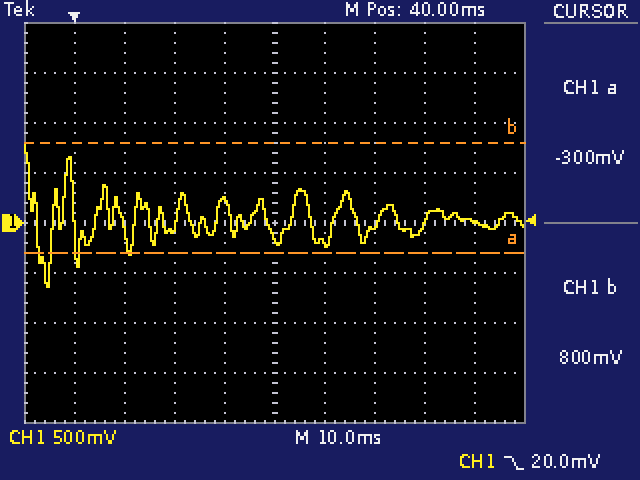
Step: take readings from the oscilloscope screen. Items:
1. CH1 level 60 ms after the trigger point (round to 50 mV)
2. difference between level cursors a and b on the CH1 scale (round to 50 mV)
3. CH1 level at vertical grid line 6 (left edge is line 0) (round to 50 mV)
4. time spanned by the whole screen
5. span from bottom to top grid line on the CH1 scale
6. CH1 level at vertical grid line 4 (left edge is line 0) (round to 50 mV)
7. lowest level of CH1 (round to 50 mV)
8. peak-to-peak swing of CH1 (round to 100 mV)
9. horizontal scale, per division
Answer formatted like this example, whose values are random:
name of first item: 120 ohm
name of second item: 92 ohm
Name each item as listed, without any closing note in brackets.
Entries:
CH1 level 60 ms after the trigger point: 0 mV
difference between level cursors a and b on the CH1 scale: 1.10 V
CH1 level at vertical grid line 6 (left edge is line 0): -200 mV
time spanned by the whole screen: 100 ms
span from bottom to top grid line on the CH1 scale: 4 V
CH1 level at vertical grid line 4 (left edge is line 0): 200 mV
lowest level of CH1: -650 mV
peak-to-peak swing of CH1: 1.40 V
horizontal scale, per division: 10 ms
